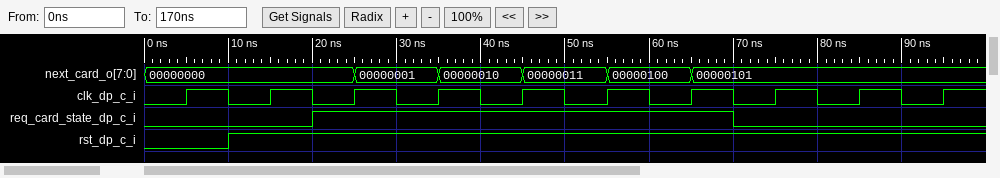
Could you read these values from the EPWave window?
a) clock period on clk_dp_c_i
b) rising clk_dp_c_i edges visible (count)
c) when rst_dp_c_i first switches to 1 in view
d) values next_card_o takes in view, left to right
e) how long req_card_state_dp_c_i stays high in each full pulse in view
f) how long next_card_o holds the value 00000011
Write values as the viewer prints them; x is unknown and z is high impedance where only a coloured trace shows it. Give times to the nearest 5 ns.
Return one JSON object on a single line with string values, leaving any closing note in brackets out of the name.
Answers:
{"clock period on clk_dp_c_i": "10 ns", "rising clk_dp_c_i edges visible": "10", "when rst_dp_c_i first switches to 1 in view": "10 ns", "values next_card_o takes in view, left to right": "00000000, 00000001, 00000010, 00000011, 00000100, 00000101", "how long req_card_state_dp_c_i stays high in each full pulse in view": "50 ns", "how long next_card_o holds the value 00000011": "10 ns"}
